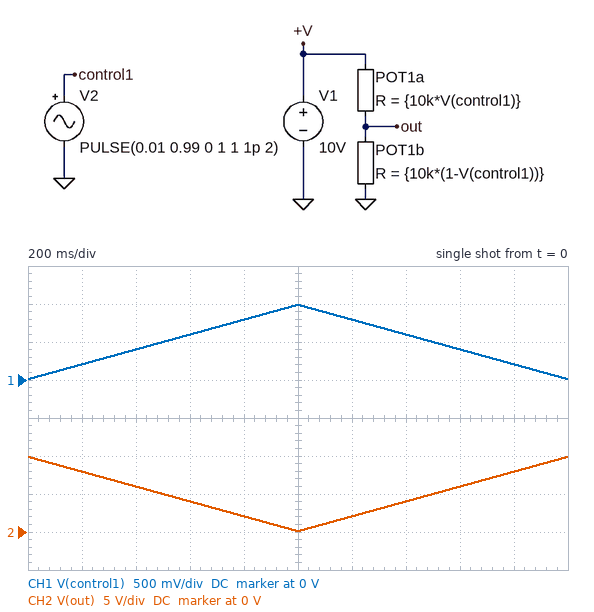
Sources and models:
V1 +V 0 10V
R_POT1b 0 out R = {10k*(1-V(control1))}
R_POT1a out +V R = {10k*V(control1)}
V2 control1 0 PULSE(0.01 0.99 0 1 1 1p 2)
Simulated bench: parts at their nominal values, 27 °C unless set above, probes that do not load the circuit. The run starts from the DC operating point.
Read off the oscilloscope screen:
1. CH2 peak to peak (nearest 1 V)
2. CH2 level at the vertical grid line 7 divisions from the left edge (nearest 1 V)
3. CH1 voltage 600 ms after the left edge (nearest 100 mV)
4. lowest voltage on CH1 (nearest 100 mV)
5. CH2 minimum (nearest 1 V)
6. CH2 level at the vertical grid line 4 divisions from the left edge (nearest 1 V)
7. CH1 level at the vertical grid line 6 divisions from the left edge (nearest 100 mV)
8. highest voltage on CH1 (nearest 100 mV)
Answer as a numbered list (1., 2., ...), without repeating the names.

1. 10 V
2. 4 V
3. 600 mV
4. 0 V
5. 0 V
6. 2 V
7. 800 mV
8. 1.0 V
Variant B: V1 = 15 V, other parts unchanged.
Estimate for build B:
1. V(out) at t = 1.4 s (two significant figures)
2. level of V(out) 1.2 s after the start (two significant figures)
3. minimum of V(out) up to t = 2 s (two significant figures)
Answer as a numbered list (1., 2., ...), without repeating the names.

1. 6.0 V
2. 3.1 V
3. 150 mV
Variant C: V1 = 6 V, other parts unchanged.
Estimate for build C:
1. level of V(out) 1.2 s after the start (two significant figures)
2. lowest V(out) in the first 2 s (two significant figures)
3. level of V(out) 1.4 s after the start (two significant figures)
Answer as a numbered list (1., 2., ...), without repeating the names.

1. 1.2 V
2. 60 mV
3. 2.4 V
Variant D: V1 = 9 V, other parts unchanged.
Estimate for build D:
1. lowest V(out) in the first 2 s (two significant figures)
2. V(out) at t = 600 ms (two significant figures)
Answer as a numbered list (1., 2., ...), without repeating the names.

1. 90 mV
2. 3.6 V
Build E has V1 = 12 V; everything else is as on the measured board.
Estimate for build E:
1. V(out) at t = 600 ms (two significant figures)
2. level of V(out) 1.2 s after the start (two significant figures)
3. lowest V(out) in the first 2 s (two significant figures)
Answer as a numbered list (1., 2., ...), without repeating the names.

1. 4.8 V
2. 2.5 V
3. 120 mV
